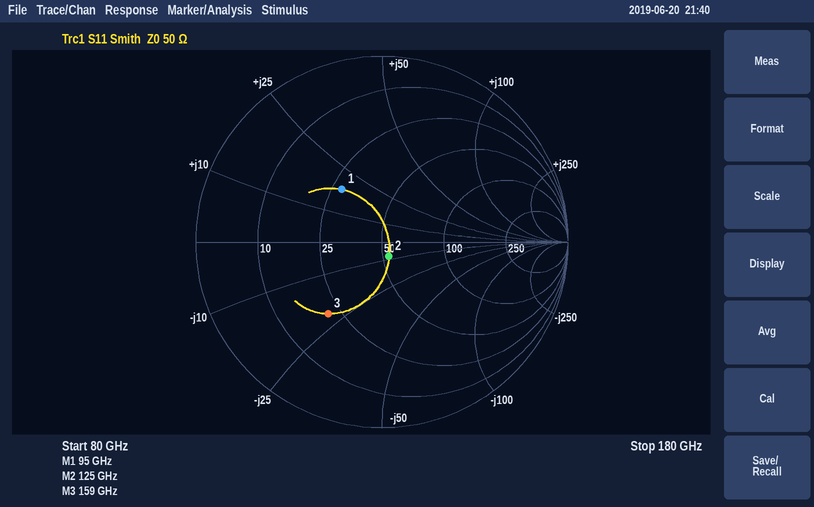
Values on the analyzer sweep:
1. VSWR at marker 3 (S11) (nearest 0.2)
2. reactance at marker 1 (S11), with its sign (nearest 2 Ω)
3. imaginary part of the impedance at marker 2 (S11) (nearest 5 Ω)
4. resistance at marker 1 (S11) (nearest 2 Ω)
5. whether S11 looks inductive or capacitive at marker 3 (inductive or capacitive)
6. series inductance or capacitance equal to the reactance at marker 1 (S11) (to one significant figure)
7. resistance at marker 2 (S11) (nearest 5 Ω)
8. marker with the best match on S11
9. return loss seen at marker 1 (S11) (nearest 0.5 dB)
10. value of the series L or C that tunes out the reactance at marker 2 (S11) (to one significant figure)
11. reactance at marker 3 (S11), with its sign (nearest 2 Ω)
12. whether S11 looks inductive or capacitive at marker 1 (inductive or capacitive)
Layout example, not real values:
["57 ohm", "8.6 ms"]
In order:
["2.8", "+18 Ω", "-10 Ω", "28 Ω", "capacitive", "30 pH", "55 Ω", "marker 2", "9.0 dB", "10 pH", "-22 Ω", "inductive"]
